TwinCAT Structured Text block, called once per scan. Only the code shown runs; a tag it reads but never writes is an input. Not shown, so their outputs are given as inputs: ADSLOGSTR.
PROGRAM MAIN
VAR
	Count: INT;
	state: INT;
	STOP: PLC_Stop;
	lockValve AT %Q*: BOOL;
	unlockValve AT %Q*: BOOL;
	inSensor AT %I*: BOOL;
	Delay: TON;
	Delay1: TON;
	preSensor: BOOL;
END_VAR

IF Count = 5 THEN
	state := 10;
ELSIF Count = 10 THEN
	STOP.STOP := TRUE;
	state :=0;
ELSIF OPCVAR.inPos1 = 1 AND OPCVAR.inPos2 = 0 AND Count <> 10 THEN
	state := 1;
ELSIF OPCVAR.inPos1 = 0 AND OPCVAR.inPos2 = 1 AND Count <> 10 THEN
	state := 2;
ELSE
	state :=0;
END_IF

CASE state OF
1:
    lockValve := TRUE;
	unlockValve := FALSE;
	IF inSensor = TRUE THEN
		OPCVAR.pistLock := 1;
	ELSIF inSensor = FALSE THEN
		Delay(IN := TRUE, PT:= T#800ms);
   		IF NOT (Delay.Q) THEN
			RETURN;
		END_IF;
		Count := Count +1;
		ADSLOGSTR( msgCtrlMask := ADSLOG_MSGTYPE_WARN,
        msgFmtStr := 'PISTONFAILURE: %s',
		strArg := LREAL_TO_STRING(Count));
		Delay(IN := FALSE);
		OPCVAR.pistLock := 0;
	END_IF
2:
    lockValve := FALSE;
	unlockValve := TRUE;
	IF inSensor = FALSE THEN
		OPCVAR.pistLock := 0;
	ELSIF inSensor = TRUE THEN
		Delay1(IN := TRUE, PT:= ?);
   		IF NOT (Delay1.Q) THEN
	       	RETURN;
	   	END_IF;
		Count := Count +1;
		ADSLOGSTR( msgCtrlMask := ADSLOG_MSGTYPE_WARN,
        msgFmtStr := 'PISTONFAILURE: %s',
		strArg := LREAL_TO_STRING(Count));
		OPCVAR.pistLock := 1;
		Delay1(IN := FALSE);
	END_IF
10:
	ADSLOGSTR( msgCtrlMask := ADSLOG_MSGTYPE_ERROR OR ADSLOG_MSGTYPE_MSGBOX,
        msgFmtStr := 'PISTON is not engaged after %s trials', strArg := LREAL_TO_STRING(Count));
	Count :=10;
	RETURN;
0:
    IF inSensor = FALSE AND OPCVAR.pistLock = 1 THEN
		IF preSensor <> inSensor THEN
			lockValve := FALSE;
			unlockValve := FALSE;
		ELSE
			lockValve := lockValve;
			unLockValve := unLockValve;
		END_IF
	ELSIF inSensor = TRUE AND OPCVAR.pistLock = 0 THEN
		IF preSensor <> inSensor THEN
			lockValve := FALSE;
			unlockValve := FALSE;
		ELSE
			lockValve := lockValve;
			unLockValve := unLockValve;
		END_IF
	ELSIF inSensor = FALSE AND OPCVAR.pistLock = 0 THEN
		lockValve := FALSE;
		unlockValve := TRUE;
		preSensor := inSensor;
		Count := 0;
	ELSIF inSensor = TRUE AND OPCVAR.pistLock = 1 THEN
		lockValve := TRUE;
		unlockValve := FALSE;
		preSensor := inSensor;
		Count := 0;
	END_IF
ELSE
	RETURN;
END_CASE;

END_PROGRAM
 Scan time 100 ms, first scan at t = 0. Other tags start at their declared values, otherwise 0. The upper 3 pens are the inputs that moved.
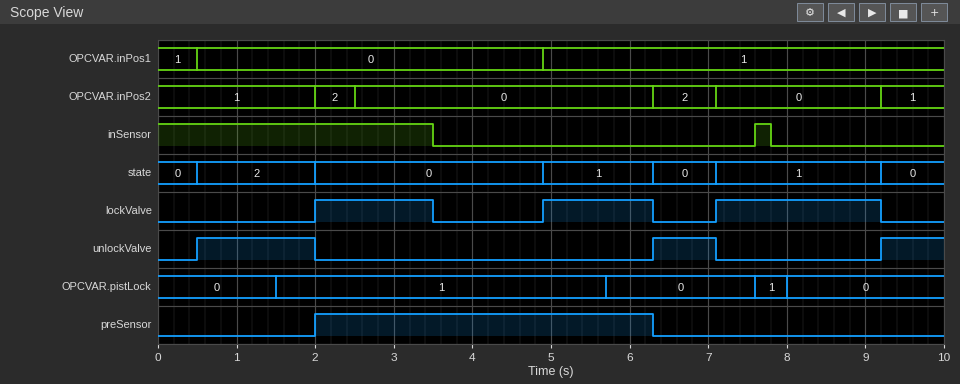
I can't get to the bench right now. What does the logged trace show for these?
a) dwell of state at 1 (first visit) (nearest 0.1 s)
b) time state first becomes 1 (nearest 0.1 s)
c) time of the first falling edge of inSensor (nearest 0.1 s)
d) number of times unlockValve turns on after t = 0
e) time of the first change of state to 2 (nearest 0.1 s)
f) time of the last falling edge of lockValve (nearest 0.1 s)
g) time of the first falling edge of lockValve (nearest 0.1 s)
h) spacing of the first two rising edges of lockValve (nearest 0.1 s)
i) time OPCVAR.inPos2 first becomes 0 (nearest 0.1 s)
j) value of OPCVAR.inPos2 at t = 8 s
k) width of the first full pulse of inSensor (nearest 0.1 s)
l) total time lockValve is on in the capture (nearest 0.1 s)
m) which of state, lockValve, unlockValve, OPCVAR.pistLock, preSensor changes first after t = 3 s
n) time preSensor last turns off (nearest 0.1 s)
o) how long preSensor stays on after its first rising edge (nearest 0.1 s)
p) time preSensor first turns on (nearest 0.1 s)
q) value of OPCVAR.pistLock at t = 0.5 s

1.4 s
4.9 s
3.5 s
3
0.5 s
9.2 s
3.5 s
2.9 s
2.5 s
0
0.2 s
5.0 s
lockValve
6.3 s
4.3 s
2.0 s
0
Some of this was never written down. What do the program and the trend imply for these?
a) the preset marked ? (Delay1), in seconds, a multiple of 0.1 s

1.0 s
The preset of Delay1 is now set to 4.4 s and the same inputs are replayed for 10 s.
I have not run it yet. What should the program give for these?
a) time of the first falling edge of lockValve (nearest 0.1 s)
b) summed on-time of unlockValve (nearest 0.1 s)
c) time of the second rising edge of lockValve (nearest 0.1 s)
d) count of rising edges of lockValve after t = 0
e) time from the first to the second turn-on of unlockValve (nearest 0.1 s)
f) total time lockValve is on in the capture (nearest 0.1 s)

6.3 s
4.5 s
7.1 s
2
3.0 s
3.5 s
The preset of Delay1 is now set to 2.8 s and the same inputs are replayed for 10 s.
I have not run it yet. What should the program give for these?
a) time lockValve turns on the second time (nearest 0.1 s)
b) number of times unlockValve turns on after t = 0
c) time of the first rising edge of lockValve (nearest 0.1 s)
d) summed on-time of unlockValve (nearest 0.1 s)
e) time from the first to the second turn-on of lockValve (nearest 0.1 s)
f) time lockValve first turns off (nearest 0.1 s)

7.1 s
4
4.9 s
4.5 s
2.2 s
6.3 s
